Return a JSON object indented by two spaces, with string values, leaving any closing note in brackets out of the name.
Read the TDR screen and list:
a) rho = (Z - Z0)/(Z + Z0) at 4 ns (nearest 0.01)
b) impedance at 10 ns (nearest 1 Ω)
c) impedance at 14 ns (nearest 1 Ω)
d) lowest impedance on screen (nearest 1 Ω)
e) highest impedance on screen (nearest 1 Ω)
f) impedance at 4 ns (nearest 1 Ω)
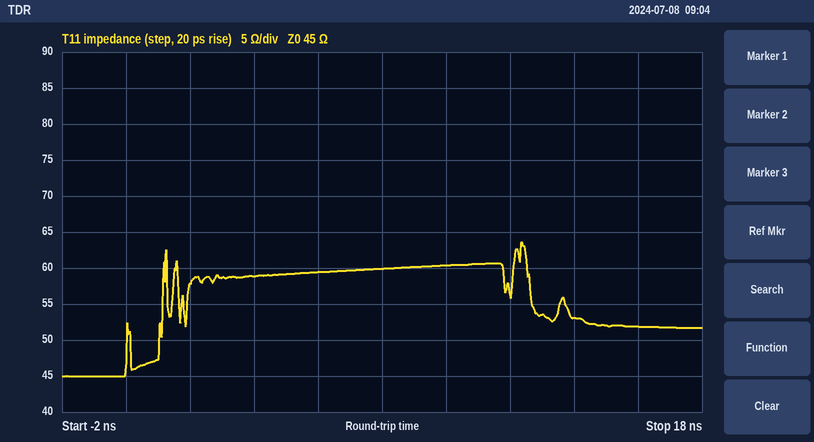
{
  "rho = (Z - Z0)/(Z + Z0) at 4 ns": "+0.13",
  "impedance at 10 ns": "60 Ω",
  "impedance at 14 ns": "53 Ω",
  "lowest impedance on screen": "45 Ω",
  "highest impedance on screen": "64 Ω",
  "impedance at 4 ns": "59 Ω"
}
